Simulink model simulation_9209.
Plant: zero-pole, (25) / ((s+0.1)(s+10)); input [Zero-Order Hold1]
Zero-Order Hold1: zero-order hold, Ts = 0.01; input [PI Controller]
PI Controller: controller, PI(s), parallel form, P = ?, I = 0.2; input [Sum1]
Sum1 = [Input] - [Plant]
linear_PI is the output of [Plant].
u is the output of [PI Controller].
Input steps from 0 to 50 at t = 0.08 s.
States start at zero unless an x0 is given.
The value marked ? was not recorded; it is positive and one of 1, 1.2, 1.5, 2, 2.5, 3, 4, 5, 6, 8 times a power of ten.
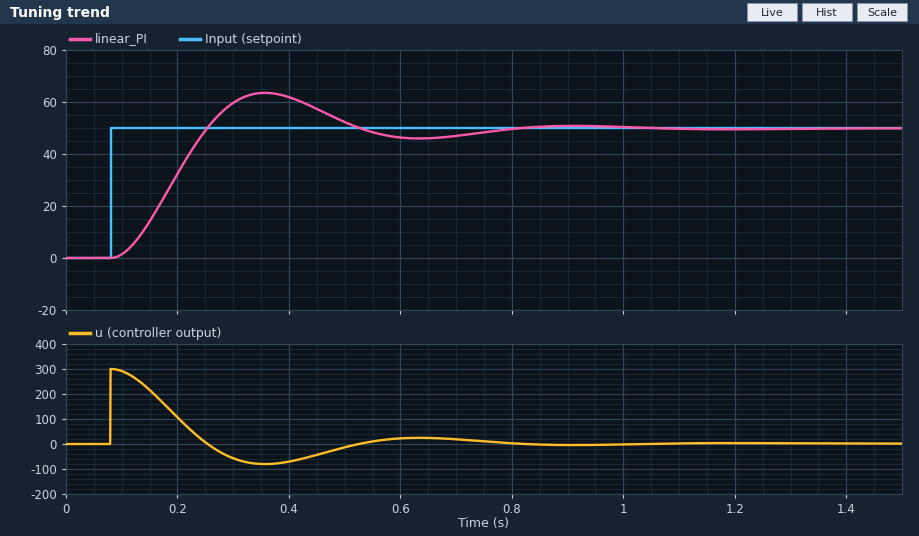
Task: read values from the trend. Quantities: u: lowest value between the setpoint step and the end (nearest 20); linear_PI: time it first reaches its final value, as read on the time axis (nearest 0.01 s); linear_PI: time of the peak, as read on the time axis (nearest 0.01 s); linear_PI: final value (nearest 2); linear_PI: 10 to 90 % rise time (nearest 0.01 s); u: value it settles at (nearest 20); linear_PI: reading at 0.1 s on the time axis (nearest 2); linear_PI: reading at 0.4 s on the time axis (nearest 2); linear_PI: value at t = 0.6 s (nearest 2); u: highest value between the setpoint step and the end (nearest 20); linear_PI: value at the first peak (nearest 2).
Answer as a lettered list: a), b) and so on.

a) -80
b) 0.25 s
c) 0.36 s
d) 50
e) 0.12 s
f) 0
g) 2
h) 62
i) 46
j) 300
k) 64
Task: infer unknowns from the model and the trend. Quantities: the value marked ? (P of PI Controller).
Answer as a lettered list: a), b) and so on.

a) 6
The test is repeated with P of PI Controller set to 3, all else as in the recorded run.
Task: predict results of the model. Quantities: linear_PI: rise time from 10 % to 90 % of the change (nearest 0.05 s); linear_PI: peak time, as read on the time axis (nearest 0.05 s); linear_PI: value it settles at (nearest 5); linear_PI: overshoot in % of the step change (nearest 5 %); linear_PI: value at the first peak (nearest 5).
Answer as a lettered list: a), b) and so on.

a) 0.20 s
b) 0.50 s
c) 50
d) 10 %
e) 55
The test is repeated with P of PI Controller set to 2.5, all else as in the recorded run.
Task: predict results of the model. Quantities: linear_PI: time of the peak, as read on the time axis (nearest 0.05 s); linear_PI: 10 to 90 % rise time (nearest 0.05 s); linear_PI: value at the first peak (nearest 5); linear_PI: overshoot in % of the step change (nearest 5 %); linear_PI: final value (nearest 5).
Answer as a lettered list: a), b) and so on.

a) 0.60 s
b) 0.25 s
c) 55
d) 10 %
e) 50
